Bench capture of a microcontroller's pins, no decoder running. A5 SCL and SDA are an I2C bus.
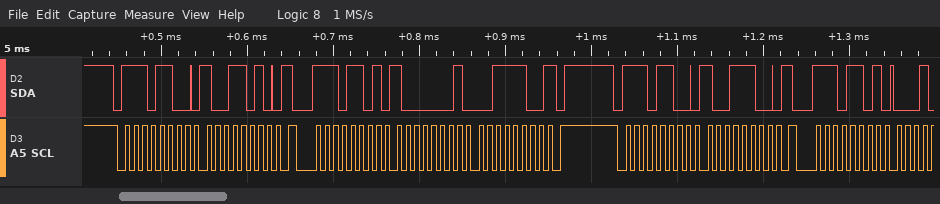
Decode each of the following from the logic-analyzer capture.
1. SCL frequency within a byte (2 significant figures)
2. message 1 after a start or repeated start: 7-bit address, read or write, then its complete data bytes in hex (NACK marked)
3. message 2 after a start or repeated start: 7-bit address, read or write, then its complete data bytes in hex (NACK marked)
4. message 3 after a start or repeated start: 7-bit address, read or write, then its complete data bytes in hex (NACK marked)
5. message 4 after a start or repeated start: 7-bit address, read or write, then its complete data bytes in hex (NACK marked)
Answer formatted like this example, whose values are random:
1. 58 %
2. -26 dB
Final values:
1. 100 kHz
2. 0x76 write: 9A
3. 0x76 read: 81 3C NACK
4. 0x76 write: 9C
5. 0x76 read
